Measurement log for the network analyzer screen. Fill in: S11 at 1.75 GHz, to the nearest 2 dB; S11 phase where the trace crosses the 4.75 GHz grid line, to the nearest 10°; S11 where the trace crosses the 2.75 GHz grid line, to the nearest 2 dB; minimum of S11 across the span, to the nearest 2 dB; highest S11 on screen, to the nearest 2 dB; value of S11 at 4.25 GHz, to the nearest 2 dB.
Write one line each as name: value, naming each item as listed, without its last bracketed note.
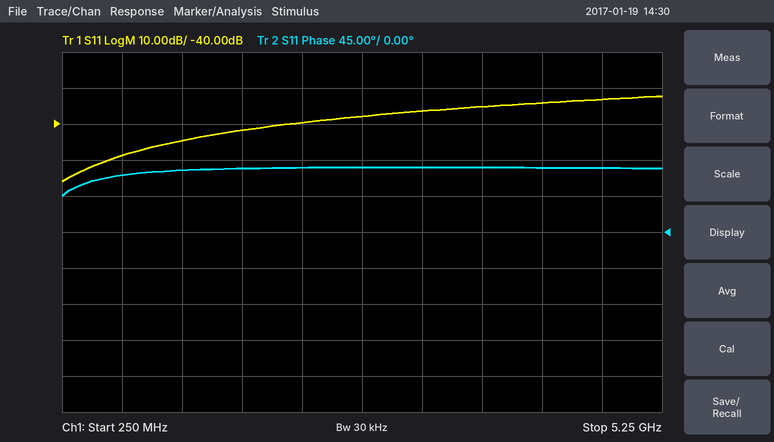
S11 at 1.75 GHz, to the nearest 2 dB: -42 dB
S11 phase where the trace crosses the 4.75 GHz grid line, to the nearest 10°: 80°
S11 where the trace crosses the 2.75 GHz grid line, to the nearest 2 dB: -38 dB
minimum of S11 across the span, to the nearest 2 dB: -56 dB
highest S11 on screen, to the nearest 2 dB: -32 dB
value of S11 at 4.25 GHz, to the nearest 2 dB: -34 dB
